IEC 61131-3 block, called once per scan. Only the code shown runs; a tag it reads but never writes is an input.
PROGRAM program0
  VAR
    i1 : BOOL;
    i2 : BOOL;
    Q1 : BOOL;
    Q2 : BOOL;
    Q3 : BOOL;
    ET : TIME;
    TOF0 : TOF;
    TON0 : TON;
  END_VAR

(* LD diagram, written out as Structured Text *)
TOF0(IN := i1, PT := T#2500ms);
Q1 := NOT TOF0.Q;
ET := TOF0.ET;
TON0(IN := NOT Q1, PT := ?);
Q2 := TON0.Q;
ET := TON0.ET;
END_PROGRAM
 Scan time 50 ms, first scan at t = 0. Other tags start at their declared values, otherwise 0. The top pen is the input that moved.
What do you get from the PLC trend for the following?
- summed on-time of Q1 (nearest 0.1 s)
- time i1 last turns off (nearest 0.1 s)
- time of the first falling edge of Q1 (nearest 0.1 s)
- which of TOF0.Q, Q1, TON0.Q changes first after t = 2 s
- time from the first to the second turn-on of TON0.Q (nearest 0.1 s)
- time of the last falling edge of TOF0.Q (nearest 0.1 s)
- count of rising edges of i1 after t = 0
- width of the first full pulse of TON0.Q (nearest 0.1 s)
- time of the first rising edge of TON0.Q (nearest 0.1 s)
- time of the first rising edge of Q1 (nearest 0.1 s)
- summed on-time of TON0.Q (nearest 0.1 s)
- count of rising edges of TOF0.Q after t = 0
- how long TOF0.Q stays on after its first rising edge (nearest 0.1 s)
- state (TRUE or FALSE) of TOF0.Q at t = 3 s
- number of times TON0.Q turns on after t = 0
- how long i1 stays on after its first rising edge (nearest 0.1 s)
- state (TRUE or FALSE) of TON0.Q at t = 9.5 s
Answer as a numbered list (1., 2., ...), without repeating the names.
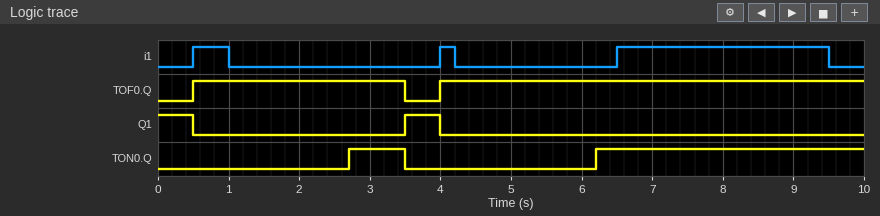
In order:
1. 1.0 s
2. 9.5 s
3. 0.5 s
4. TON0.Q
5. 3.5 s
6. 3.5 s
7. 3
8. 0.8 s
9. 2.7 s
10. 3.5 s
11. 4.6 s
12. 2
13. 3.0 s
14. TRUE
15. 2
16. 0.5 s
17. TRUE
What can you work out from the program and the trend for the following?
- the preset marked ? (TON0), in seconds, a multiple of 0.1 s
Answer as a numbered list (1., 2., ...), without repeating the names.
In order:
1. 2.2 s
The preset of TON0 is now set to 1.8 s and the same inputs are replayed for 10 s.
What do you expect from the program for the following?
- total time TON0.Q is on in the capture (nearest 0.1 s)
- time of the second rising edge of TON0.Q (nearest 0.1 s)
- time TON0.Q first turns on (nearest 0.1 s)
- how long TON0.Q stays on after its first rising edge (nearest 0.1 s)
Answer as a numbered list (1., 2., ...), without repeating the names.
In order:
1. 5.4 s
2. 5.8 s
3. 2.3 s
4. 1.2 s
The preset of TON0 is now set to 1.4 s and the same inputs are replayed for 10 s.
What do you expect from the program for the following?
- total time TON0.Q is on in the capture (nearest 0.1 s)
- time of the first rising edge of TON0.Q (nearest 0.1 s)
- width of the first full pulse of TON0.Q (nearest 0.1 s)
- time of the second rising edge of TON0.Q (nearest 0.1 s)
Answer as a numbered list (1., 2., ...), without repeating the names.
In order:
1. 6.2 s
2. 1.9 s
3. 1.6 s
4. 5.4 s
